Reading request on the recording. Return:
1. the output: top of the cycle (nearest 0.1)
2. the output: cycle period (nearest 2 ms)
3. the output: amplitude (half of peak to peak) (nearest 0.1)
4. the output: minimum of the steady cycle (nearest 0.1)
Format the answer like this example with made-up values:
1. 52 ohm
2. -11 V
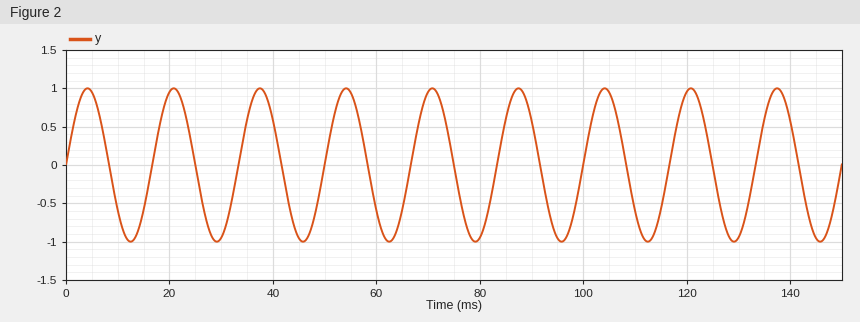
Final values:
1. 1.0
2. 16 ms
3. 1.0
4. -1.0
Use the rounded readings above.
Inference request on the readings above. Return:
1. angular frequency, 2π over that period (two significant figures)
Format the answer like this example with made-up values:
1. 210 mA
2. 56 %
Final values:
1. 0.39 rad/ms
